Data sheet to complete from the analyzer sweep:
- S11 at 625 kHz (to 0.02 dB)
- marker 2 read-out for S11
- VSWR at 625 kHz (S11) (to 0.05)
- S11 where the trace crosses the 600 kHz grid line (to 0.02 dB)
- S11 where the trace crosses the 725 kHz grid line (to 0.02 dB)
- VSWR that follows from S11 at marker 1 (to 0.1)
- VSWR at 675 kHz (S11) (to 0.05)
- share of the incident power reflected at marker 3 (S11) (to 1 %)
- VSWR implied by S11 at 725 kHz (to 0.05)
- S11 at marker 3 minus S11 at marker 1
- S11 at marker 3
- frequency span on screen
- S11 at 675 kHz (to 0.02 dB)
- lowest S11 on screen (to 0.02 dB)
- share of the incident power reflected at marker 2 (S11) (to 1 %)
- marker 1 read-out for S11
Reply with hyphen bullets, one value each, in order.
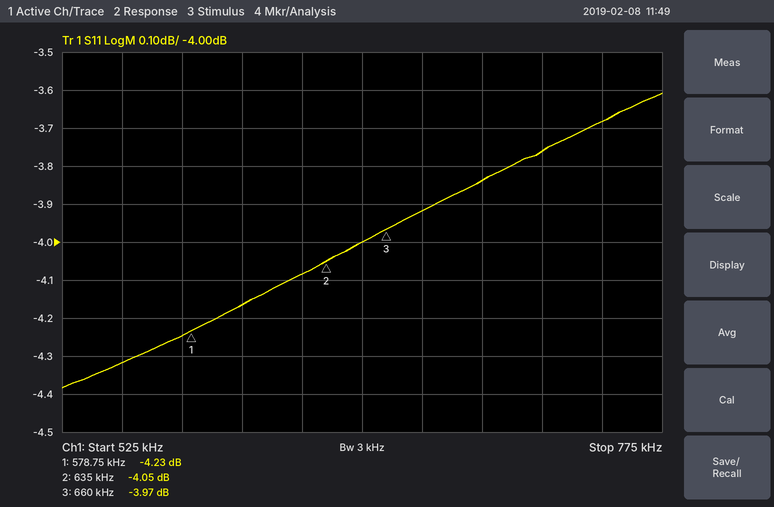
- -4.08 dB
- -4.05 dB
- 4.35
- -4.16 dB
- -3.76 dB
- 4.2
- 4.50
- 40 %
- 4.70
- 0.26 dB
- -3.97 dB
- 250 kHz
- -3.92 dB
- -4.38 dB
- 39 %
- -4.23 dB
